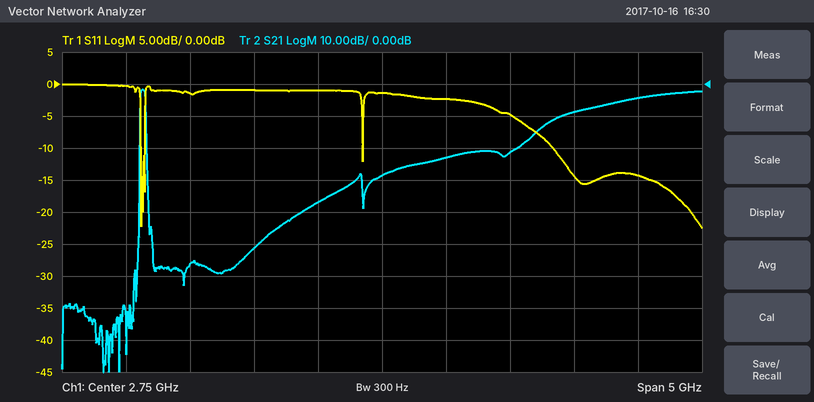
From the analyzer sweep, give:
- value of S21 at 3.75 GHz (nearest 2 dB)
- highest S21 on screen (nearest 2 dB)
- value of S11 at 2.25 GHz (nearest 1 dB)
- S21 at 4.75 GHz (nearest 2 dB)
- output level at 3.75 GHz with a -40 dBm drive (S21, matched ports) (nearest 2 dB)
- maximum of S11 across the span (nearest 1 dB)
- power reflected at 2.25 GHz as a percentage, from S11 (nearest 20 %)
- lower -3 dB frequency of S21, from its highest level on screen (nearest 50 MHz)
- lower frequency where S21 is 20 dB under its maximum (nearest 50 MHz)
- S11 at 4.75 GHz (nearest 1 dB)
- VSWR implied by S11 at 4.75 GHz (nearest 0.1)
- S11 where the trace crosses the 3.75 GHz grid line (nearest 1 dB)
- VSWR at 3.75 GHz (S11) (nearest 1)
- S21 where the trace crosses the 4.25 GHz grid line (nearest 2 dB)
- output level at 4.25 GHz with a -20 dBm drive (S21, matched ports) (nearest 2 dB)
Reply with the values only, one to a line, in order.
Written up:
-22 dB
-2 dB
-1 dB
-4 dB
-62 dBm
0 dB
80 %
850 MHz
850 MHz
-14 dB
1.5
-5 dB
4
-8 dB
-28 dBm
